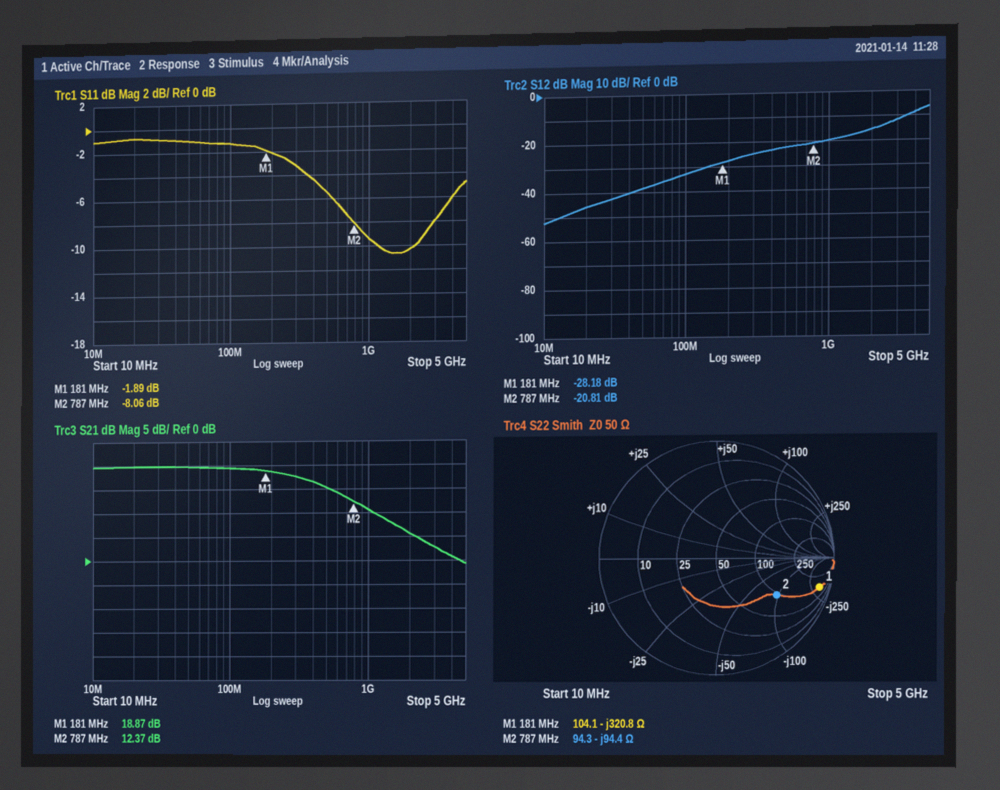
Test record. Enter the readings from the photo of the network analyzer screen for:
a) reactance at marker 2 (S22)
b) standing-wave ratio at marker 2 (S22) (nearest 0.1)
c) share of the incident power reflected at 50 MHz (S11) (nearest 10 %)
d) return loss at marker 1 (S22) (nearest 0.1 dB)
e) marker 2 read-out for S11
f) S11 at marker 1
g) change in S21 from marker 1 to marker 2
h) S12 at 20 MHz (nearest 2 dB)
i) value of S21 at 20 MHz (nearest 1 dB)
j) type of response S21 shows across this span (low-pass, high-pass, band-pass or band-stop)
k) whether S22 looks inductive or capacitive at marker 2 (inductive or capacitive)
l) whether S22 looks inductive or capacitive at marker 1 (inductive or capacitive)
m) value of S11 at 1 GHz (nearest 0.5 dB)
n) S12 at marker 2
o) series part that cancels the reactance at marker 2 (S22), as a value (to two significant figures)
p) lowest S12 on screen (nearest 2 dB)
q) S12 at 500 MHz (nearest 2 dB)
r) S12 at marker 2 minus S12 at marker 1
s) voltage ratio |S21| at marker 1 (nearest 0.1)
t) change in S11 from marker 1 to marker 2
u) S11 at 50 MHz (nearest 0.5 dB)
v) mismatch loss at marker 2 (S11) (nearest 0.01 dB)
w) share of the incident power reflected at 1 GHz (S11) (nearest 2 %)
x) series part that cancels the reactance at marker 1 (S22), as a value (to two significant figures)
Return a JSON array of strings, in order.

["-94.4 Ω", "4.1", "80 %", "0.8 dB", "-8.06 dB", "-1.89 dB", "-6.50 dB", "-46 dB", "20 dB", "low-pass", "capacitive", "capacitive", "-9.5 dB", "-20.81 dB", "19 nH", "-52 dB", "-22 dB", "7.37 dB", "8.8", "-6.17 dB", "-1.0 dB", "0.74 dB", "12 %", "280 nH"]
